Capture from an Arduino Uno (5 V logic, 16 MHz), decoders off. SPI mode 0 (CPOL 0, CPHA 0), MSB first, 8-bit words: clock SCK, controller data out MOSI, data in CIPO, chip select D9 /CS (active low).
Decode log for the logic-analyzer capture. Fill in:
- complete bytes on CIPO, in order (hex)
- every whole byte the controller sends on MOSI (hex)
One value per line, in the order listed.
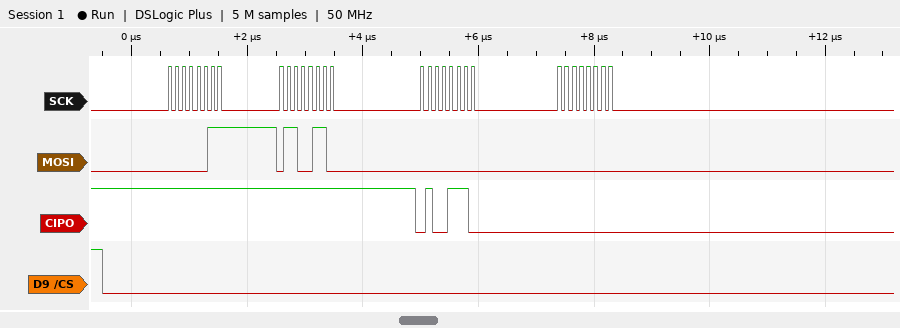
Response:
FF FF 4E 00
03 66 00 00
